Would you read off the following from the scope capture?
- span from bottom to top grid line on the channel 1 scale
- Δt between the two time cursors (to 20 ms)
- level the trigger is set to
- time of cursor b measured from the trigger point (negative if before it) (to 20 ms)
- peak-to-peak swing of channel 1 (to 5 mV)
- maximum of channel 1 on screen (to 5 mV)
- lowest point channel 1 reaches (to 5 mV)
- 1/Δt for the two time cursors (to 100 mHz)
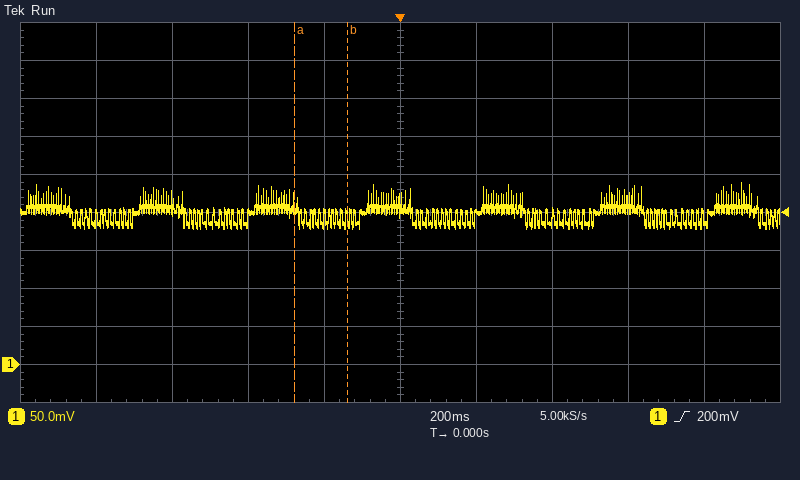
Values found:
500 mV
140 ms
200 mV
-140 ms
60 mV
240 mV
180 mV
7.1 Hz
